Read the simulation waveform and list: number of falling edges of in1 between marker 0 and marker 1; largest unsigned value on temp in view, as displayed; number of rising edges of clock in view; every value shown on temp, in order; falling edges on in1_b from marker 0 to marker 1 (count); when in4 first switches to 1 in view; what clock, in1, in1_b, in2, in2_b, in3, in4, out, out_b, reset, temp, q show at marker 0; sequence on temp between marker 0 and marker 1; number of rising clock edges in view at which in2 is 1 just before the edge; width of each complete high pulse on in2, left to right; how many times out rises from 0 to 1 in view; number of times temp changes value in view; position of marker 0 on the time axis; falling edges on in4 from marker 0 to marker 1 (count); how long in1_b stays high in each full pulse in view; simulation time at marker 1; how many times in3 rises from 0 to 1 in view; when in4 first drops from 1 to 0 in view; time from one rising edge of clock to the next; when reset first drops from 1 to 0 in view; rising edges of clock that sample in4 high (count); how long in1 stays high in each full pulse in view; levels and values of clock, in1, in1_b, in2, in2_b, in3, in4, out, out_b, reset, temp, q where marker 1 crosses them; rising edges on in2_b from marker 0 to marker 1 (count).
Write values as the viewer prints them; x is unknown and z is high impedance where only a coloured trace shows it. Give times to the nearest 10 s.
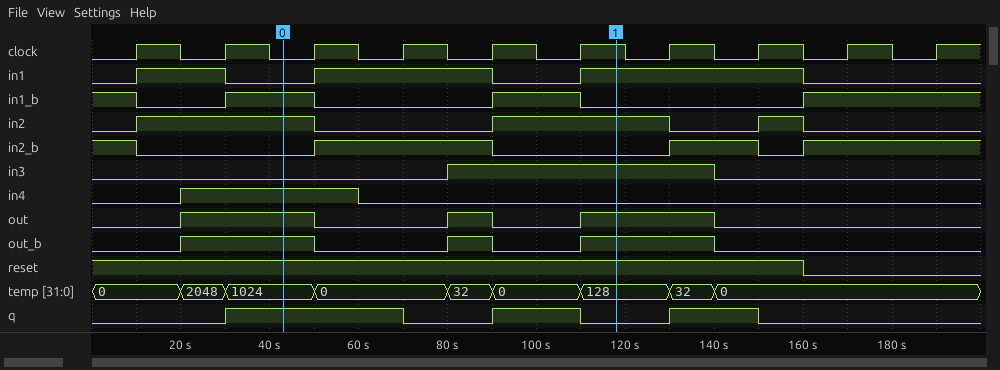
1
2048
10
0, 2048, 1024, 0, 32, 0, 128, 32, 0
2
20 s
clock=0, in1=0, in1_b=1, in2=1, in2_b=0, in3=0, in4=1, out=1, out_b=1, reset=1, temp=1024, q=1
1024, 0, 32, 0, 128
4
40 s, 40 s, 10 s
3
8
40 s
1
20 s, 20 s
120 s
1
60 s
20 s
160 s
2
20 s, 40 s, 50 s
clock=1, in1=1, in1_b=0, in2=1, in2_b=0, in3=1, in4=0, out=1, out_b=1, reset=1, temp=128, q=0
1
